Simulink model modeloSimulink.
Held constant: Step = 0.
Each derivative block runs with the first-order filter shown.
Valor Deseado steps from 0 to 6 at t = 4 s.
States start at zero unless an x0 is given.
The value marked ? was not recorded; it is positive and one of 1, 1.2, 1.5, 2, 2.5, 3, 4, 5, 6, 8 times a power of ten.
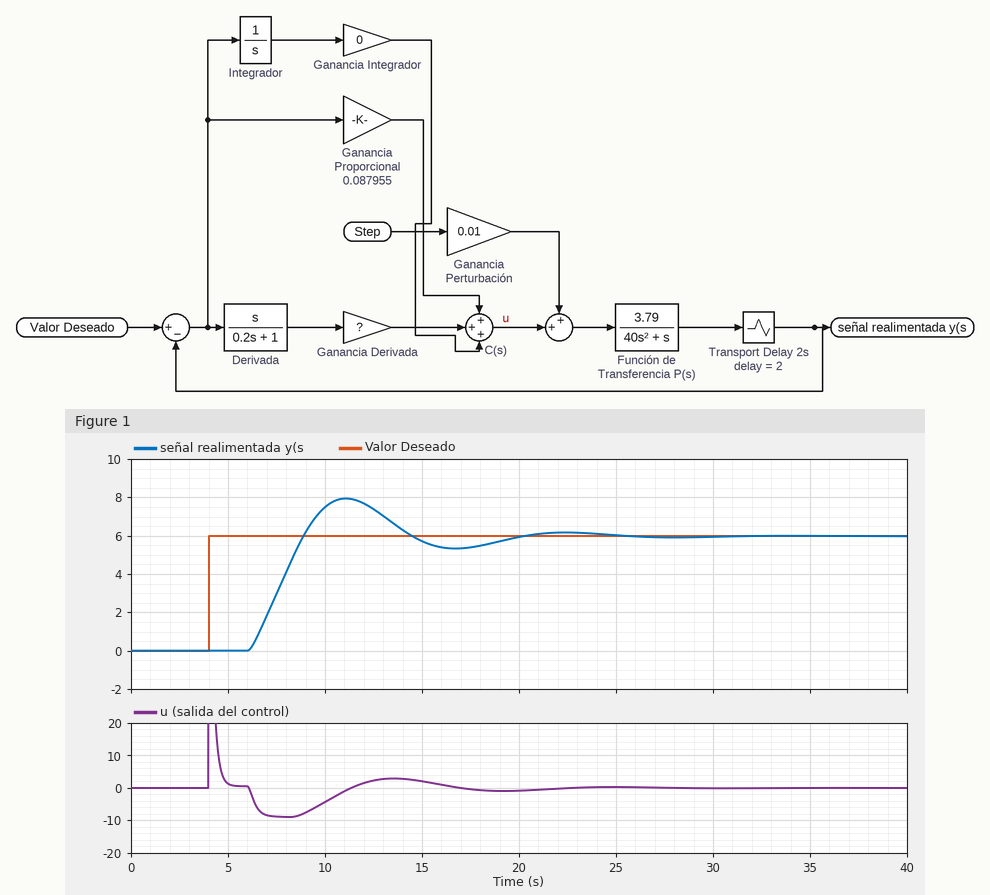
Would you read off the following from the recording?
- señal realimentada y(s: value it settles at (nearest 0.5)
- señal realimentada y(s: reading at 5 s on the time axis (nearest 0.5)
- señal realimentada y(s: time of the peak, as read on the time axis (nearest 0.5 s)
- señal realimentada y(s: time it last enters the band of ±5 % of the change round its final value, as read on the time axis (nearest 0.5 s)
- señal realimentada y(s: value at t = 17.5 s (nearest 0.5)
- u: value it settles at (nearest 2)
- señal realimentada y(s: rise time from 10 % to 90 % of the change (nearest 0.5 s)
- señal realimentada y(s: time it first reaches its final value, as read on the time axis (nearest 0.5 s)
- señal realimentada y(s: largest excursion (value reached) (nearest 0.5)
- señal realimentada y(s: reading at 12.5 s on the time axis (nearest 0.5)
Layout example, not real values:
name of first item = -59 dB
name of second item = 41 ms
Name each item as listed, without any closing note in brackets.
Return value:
señal realimentada y(s: value it settles at = 6.0
señal realimentada y(s: reading at 5 s on the time axis = 0.0
señal realimentada y(s: time of the peak, as read on the time axis = 11.0 s
señal realimentada y(s: time it last enters the band of ±5 % of the change round its final value, as read on the time axis = 19.0 s
señal realimentada y(s: value at t = 17.5 s = 5.5
u: value it settles at = 0
señal realimentada y(s: rise time from 10 % to 90 % of the change = 2.0 s
señal realimentada y(s: time it first reaches its final value, as read on the time axis = 9.0 s
señal realimentada y(s: largest excursion (value reached) = 8.0
señal realimentada y(s: reading at 12.5 s on the time axis = 7.5
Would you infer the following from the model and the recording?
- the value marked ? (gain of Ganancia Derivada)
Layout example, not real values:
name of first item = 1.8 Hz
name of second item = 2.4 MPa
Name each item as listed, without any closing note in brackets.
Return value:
the value marked ? = 4
